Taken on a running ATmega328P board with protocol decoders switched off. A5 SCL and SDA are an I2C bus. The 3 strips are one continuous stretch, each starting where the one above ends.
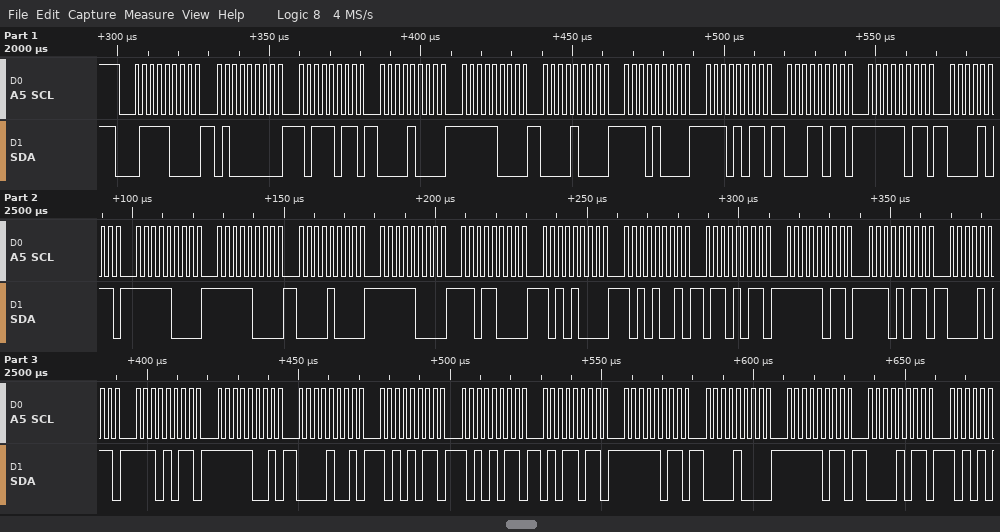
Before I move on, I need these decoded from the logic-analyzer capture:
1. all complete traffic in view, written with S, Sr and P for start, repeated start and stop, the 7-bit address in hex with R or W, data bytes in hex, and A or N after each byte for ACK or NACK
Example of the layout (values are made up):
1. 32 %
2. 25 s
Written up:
1. S 3CW A 40 A BB A 08 A F8 A 08 A E8 A EB A 1B A FB A 0B A F8 A F8 A 08 A F8 A D8 A A8 A A9 A 6B A FB A EB A 0B A EB A F9 A 09 A AB A AB A 5B A FB A 08 A FB A 0B A
